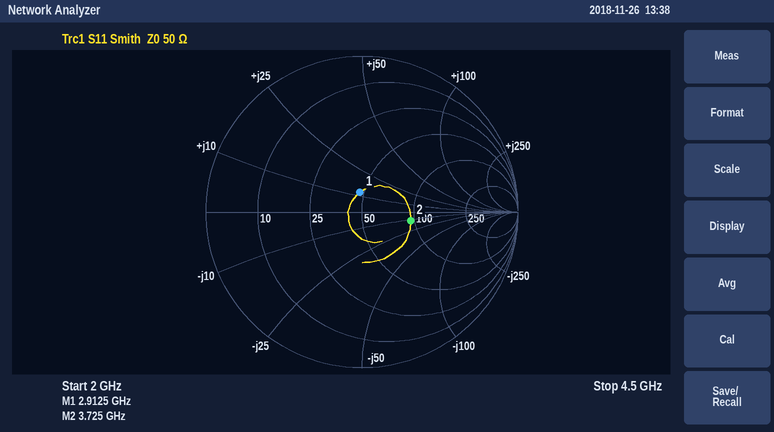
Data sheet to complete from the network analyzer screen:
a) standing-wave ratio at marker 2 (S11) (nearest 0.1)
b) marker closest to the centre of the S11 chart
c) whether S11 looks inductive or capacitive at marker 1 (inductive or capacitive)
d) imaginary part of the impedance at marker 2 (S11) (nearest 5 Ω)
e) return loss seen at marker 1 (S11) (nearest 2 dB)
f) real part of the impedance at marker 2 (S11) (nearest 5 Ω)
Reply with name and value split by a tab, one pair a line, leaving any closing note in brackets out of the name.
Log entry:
standing-wave ratio at marker 2 (S11)	1.9
marker closest to the centre of the S11 chart	marker 1
whether S11 looks inductive or capacitive at marker 1	inductive
imaginary part of the impedance at marker 2 (S11)	-10 Ω
return loss seen at marker 1 (S11)	18 dB
real part of the impedance at marker 2 (S11)	95 Ω
